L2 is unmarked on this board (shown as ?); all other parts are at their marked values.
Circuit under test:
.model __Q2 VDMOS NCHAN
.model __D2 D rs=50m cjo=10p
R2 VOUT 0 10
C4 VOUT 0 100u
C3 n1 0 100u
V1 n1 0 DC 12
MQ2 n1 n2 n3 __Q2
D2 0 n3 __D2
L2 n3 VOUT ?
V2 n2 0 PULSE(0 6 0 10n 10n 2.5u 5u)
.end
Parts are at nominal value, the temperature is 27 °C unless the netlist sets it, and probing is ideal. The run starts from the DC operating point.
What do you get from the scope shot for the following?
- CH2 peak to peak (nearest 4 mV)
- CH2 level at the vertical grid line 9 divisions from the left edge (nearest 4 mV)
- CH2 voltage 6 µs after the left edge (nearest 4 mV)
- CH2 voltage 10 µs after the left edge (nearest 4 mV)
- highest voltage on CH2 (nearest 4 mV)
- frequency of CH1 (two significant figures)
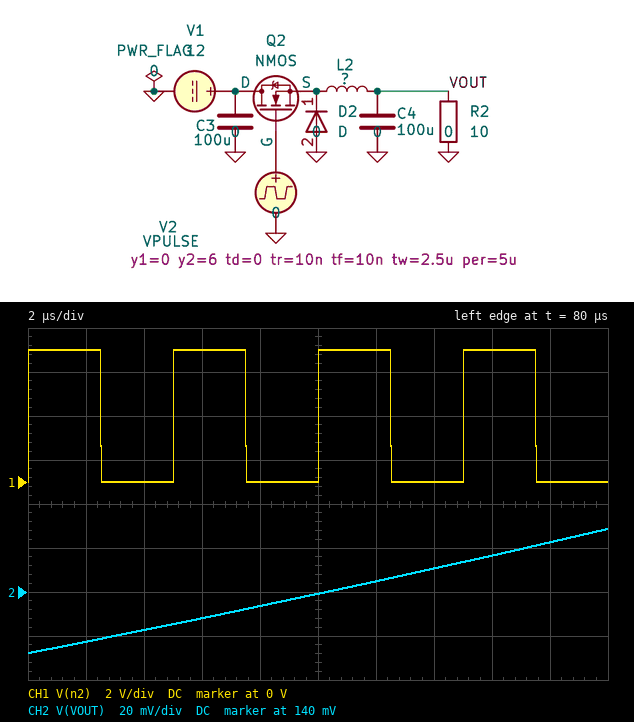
56 mV
164 mV
128 mV
140 mV
168 mV
200 kHz
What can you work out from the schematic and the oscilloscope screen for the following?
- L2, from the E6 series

330 µH
